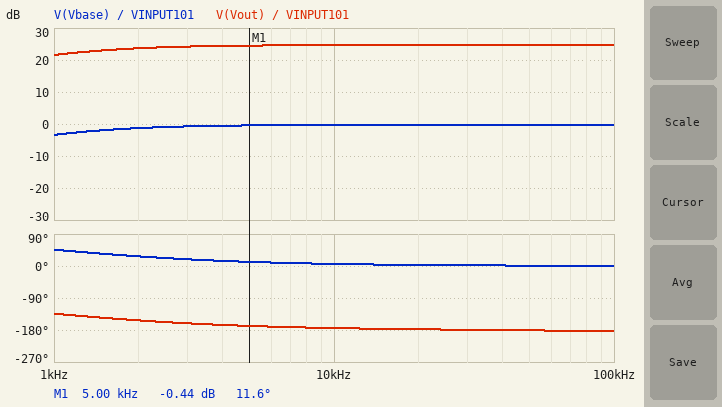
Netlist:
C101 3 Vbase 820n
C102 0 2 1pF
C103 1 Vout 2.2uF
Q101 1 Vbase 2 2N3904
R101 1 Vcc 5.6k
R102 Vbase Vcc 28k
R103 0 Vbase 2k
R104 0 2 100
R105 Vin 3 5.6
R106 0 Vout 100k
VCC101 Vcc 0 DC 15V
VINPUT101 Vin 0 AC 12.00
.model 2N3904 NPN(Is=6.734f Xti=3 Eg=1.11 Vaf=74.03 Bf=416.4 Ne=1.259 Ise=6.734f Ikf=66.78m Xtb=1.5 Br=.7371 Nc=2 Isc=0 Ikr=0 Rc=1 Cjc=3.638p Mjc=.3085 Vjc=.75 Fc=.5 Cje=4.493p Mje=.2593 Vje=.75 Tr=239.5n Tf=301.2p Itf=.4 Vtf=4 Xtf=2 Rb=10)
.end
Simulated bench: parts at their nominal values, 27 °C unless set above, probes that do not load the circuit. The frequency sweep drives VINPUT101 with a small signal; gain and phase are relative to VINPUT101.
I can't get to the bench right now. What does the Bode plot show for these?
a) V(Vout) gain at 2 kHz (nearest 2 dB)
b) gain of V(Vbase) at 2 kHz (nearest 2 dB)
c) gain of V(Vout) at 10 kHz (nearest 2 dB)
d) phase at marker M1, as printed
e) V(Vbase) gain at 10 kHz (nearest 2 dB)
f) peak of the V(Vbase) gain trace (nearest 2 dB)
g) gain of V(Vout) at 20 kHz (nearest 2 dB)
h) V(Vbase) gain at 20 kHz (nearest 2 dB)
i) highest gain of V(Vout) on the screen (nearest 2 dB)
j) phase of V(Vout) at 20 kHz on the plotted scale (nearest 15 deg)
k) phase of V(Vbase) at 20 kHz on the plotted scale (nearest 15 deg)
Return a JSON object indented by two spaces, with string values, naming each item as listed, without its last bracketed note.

{
  "V(Vout) gain at 2 kHz": "24 dB",
  "gain of V(Vbase) at 2 kHz": "-2 dB",
  "gain of V(Vout) at 10 kHz": "24 dB",
  "phase at marker M1, as printed": "11.6 deg",
  "V(Vbase) gain at 10 kHz": "0 dB",
  "peak of the V(Vbase) gain trace": "0 dB",
  "gain of V(Vout) at 20 kHz": "24 dB",
  "V(Vbase) gain at 20 kHz": "0 dB",
  "highest gain of V(Vout) on the screen": "24 dB",
  "phase of V(Vout) at 20 kHz on the plotted scale": "-180 deg",
  "phase of V(Vbase) at 20 kHz on the plotted scale": "0 deg"
}
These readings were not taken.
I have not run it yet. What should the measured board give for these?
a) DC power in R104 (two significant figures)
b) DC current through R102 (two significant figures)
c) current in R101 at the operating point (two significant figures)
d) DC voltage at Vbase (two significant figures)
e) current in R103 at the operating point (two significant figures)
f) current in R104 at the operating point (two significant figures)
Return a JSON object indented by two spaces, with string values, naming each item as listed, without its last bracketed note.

{
  "DC power in R104": "690 µW",
  "DC current through R102": "500 µA",
  "current in R101 at the operating point": "2.6 mA",
  "DC voltage at Vbase": "950 mV",
  "current in R103 at the operating point": "480 µA",
  "current in R104 at the operating point": "2.6 mA"
}
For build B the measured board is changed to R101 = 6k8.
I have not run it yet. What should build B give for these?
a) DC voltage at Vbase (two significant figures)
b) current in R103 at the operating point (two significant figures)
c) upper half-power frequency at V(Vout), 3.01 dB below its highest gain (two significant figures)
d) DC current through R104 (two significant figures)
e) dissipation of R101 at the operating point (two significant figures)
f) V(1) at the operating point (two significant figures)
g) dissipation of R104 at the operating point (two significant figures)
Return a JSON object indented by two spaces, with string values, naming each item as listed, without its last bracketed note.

{
  "DC voltage at Vbase": "910 mV",
  "current in R103 at the operating point": "450 µA",
  "upper half-power frequency at V(Vout), 3.01 dB below its highest gain": "1.1 MHz",
  "DC current through R104": "2.2 mA",
  "dissipation of R101 at the operating point": "32 mW",
  "V(1) at the operating point": "340 mV",
  "dissipation of R104 at the operating point": "490 µW"
}
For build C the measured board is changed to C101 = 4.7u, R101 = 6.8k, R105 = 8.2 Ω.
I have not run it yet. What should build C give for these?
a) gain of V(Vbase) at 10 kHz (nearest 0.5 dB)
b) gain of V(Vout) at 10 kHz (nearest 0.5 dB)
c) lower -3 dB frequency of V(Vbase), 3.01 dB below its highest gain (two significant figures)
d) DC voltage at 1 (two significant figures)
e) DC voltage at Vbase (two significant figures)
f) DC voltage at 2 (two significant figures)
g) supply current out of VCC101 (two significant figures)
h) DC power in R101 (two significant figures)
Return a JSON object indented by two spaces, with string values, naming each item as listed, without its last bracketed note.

{
  "gain of V(Vbase) at 10 kHz": "-0.5 dB",
  "gain of V(Vout) at 10 kHz": "12.5 dB",
  "lower -3 dB frequency of V(Vbase), 3.01 dB below its highest gain": "240 Hz",
  "DC voltage at 1": "340 mV",
  "DC voltage at Vbase": "910 mV",
  "DC voltage at 2": "220 mV",
  "supply current out of VCC101": "2.7 mA",
  "DC power in R101": "32 mW"
}
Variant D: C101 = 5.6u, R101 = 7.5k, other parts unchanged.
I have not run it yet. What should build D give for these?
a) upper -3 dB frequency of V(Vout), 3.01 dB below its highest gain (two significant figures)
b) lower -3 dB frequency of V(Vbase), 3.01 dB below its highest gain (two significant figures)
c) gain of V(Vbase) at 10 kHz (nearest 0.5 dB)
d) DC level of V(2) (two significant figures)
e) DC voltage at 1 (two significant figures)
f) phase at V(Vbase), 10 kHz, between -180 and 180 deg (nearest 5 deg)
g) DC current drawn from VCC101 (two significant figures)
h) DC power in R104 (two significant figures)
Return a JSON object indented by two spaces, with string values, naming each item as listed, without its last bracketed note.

{
  "upper -3 dB frequency of V(Vout), 3.01 dB below its highest gain": "1.1 MHz",
  "lower -3 dB frequency of V(Vbase), 3.01 dB below its highest gain": "210 Hz",
  "gain of V(Vbase) at 10 kHz": "-0.5 dB",
  "DC level of V(2)": "200 mV",
  "DC voltage at 1": "310 mV",
  "phase at V(Vbase), 10 kHz, between -180 and 180 deg": "0 deg",
  "DC current drawn from VCC101": "2.5 mA",
  "DC power in R104": "410 µW"
}
